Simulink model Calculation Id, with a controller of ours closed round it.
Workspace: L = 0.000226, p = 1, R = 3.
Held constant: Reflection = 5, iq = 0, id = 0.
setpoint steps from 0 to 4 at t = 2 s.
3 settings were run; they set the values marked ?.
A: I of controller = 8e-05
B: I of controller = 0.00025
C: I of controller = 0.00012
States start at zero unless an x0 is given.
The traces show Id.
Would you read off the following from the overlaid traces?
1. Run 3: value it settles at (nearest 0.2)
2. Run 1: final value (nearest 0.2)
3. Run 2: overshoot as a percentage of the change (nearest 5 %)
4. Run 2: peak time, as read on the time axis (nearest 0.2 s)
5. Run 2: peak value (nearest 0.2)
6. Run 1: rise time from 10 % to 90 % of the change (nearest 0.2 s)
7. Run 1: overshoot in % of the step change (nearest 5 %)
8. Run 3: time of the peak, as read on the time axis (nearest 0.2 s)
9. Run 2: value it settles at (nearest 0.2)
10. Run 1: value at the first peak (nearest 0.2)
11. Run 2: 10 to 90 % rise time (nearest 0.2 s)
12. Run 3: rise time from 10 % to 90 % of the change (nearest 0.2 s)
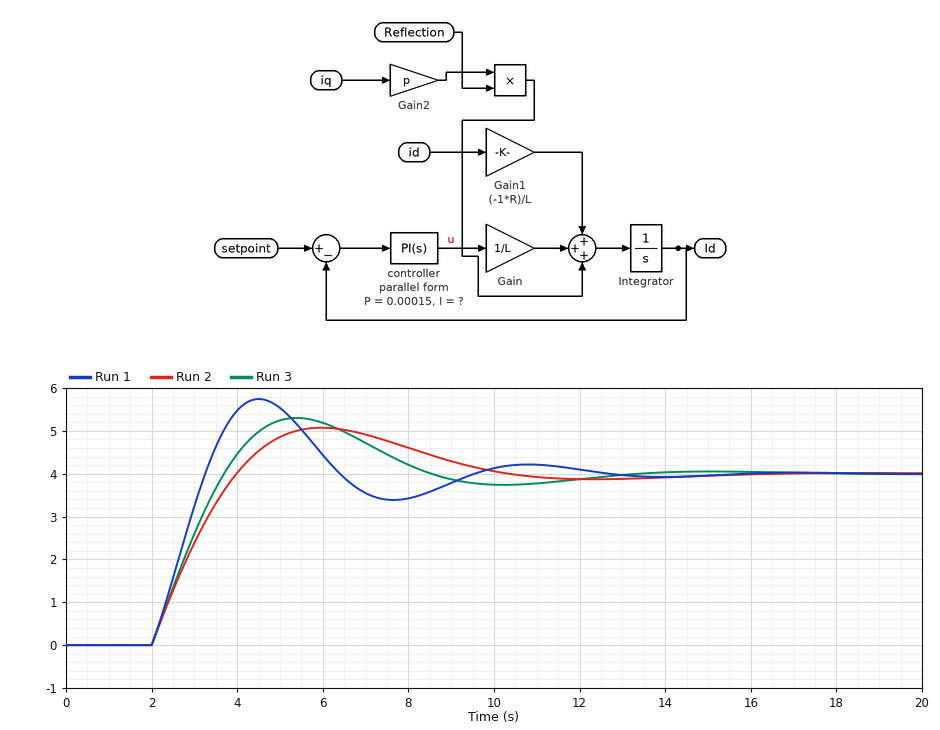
4.0
4.0
25 %
6.0 s
5.0
1.0 s
45 %
5.4 s
4.0
5.8
1.6 s
1.4 s
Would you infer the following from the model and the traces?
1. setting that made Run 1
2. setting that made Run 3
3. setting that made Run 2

B
C
A
